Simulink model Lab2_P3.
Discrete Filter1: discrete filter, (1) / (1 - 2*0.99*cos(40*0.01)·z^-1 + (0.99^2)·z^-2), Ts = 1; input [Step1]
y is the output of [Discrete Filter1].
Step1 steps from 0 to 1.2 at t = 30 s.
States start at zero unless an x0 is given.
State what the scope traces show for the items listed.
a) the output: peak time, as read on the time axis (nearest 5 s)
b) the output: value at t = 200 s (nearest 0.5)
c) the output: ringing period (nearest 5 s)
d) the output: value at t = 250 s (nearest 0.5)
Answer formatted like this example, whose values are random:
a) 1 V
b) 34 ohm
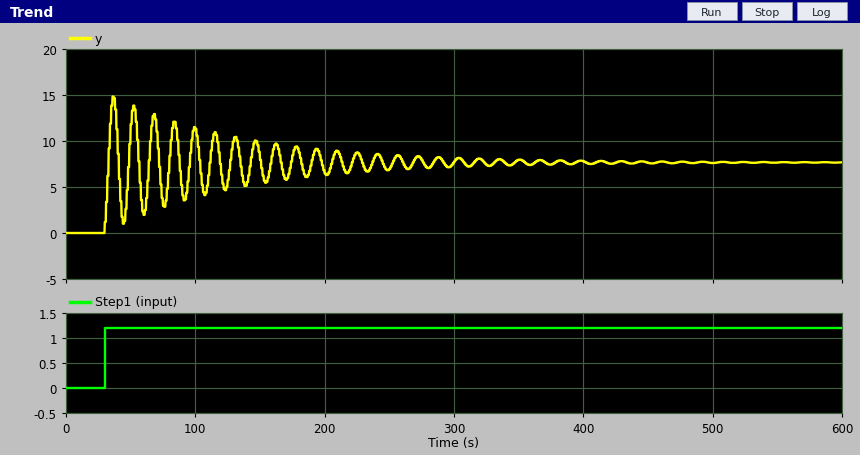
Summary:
a) 35 s
b) 6.5
c) 15 s
d) 7.0
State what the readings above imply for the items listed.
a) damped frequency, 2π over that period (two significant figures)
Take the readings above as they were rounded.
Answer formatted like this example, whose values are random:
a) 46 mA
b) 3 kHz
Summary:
a) 0.42 rad/s
